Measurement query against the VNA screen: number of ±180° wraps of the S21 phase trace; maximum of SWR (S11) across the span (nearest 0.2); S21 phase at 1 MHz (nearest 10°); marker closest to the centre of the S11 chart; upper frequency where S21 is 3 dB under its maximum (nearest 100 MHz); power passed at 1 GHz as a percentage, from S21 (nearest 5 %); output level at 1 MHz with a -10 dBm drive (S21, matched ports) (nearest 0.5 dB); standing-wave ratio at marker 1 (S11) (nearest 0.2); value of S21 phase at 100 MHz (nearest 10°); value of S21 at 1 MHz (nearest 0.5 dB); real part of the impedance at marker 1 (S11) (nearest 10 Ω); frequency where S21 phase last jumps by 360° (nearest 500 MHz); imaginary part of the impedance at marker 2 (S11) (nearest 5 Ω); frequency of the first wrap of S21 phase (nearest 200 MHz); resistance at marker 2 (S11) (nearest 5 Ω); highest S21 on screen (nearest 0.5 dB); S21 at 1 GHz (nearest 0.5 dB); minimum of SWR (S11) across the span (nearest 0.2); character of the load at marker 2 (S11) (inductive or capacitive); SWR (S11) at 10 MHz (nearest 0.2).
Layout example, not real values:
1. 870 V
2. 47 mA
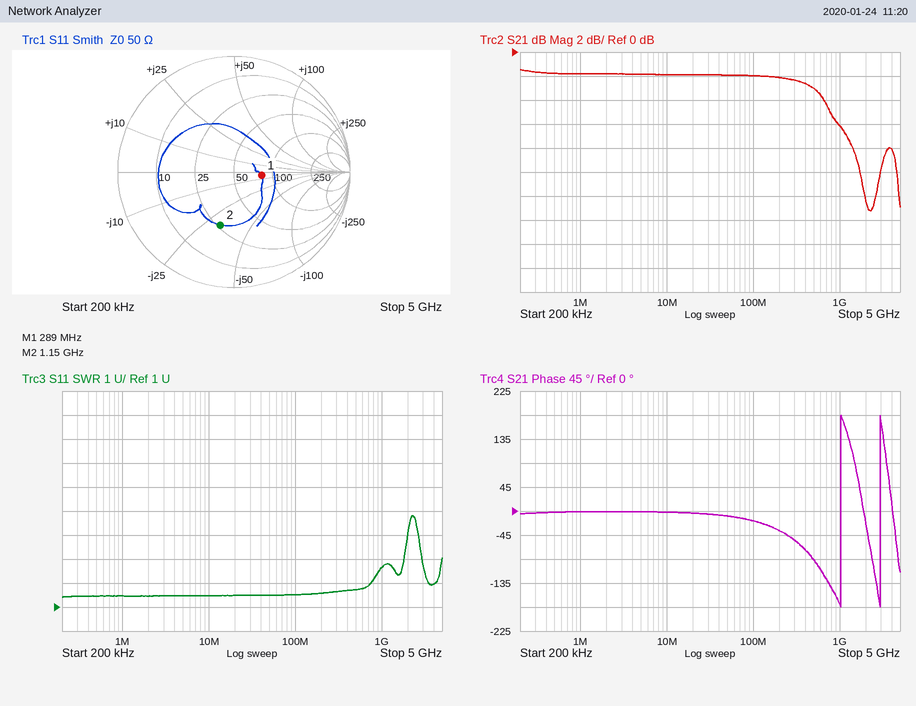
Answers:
1. 2
2. 4.8
3. 0°
4. marker 1
5. 700 MHz
6. 25 %
7. -12.0 dBm
8. 1.6
9. -20°
10. -2.0 dB
11. 80 Ω
12. 3.0 GHz
13. -30 Ω
14. 1.0 GHz
15. 25 Ω
16. -1.5 dB
17. -6.0 dB
18. 1.4
19. capacitive
20. 1.4
